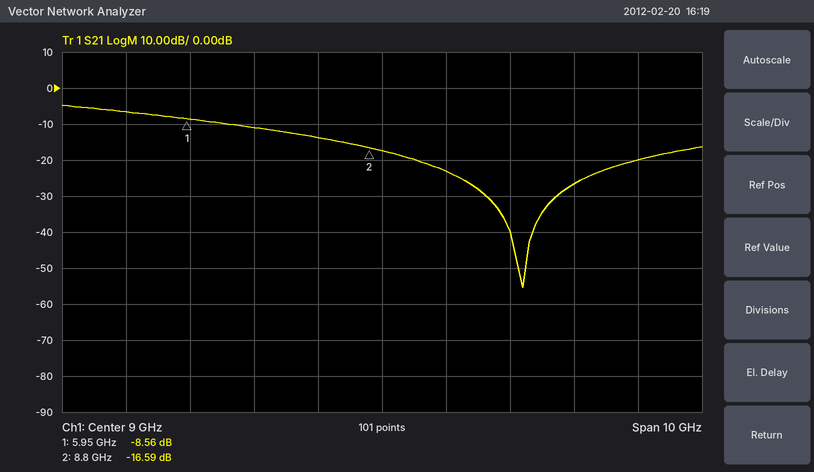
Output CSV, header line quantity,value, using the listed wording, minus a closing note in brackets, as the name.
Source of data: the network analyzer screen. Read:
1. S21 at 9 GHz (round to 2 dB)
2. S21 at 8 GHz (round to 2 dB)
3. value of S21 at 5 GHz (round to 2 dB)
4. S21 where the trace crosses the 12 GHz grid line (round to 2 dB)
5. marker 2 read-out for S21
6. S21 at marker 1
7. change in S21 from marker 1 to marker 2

quantity,value
S21 at 9 GHz,-18 dB
S21 at 8 GHz,-14 dB
value of S21 at 5 GHz,-6 dB
S21 where the trace crosses the 12 GHz grid line,-26 dB
marker 2 read-out for S21,-16.59 dB
S21 at marker 1,-8.56 dB
change in S21 from marker 1 to marker 2,-8.03 dB
